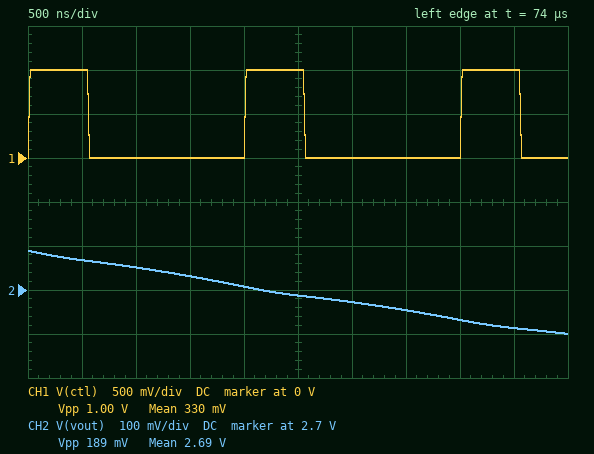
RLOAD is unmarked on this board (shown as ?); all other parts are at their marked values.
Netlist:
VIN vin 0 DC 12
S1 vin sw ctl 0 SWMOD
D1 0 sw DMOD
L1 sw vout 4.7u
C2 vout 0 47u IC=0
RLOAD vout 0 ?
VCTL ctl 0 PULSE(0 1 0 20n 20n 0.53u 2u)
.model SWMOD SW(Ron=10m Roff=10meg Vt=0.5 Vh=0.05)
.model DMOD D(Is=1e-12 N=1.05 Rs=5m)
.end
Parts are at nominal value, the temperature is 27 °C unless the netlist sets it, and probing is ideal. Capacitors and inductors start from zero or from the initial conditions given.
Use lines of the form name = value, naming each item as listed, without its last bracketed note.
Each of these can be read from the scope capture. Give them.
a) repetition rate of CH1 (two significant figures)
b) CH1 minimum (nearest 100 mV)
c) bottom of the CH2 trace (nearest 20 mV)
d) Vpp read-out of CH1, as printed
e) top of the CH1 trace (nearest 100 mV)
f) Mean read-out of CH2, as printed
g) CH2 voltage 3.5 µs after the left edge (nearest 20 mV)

repetition rate of CH1 = 500 kHz
CH1 minimum = 0 V
bottom of the CH2 trace = 2.60 V
Vpp read-out of CH1, as printed = 1.00 V
top of the CH1 trace = 1.0 V
Mean read-out of CH2, as printed = 2.69 V
CH2 voltage 3.5 µs after the left edge = 2.66 V
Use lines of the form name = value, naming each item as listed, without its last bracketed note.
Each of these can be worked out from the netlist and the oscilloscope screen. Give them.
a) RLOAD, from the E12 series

RLOAD, from the E12 series = 0.56 Ω
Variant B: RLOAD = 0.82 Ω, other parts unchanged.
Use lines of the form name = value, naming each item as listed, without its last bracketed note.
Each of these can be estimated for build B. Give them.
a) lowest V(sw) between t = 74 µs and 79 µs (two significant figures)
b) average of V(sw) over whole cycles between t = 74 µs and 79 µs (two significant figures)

lowest V(sw) between t = 74 µs and 79 µs = -760 mV
average of V(sw) over whole cycles between t = 74 µs and 79 µs = 2.8 V
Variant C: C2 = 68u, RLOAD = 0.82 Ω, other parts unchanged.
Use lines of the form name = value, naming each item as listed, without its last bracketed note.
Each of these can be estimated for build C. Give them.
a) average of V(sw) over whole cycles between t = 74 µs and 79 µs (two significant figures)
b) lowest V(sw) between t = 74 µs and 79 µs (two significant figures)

average of V(sw) over whole cycles between t = 74 µs and 79 µs = 3.5 V
lowest V(sw) between t = 74 µs and 79 µs = -760 mV
